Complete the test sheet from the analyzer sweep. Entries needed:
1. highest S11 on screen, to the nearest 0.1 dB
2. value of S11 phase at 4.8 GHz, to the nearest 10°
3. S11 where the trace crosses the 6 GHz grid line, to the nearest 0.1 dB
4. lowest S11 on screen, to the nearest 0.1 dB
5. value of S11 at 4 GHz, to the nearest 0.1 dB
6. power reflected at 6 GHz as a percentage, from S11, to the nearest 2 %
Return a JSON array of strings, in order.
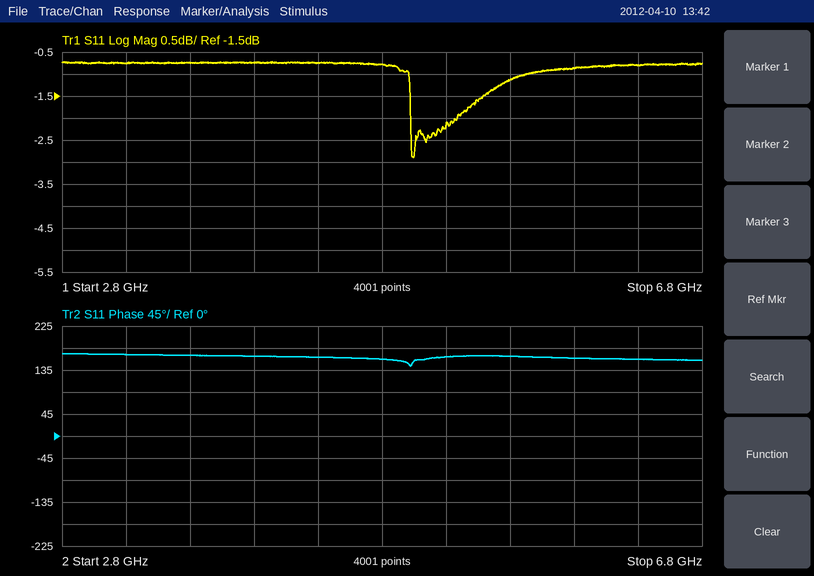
["-0.7 dB", "160°", "-0.9 dB", "-2.9 dB", "-0.7 dB", "82 %"]
